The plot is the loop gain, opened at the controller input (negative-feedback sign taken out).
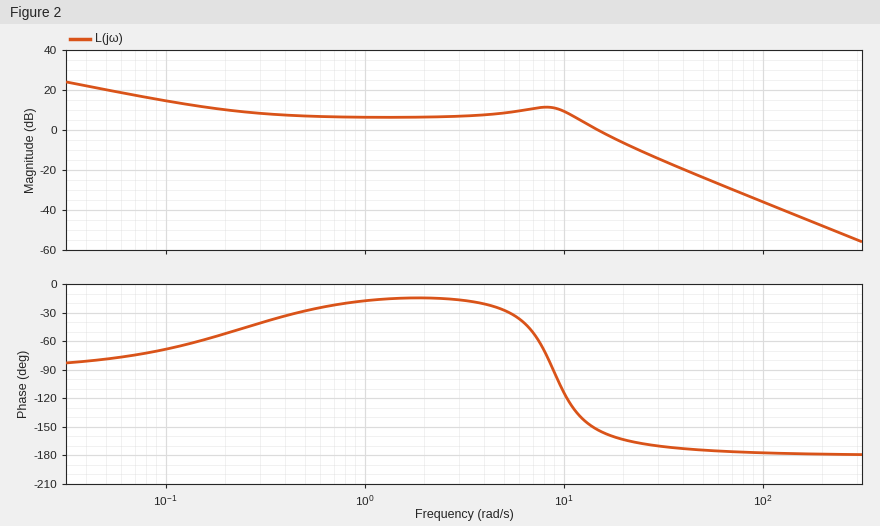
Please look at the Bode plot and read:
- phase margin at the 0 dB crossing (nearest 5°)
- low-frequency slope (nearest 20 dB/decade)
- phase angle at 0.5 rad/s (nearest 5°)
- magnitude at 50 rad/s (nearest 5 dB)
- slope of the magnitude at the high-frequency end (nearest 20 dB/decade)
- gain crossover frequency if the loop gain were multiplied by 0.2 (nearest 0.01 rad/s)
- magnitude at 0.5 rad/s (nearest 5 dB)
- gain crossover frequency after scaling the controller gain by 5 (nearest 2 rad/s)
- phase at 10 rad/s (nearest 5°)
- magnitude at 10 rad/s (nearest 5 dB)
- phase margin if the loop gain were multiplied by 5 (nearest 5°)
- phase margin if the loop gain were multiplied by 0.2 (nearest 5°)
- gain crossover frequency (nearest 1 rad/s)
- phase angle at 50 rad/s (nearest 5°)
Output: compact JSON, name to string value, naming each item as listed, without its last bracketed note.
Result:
{"phase margin at the 0 dB crossing": "25°", "low-frequency slope": "-20 dB/decade", "phase angle at 0.5 rad/s": "-30°", "magnitude at 50 rad/s": "-25 dB", "slope of the magnitude at the high-frequency end": "-40 dB/decade", "gain crossover frequency if the loop gain were multiplied by 0.2": "0.11 rad/s", "magnitude at 0.5 rad/s": "5 dB", "gain crossover frequency after scaling the controller gain by 5": "30 rad/s", "phase at 10 rad/s": "-115°", "magnitude at 10 rad/s": "10 dB", "phase margin if the loop gain were multiplied by 5": "10°", "phase margin if the loop gain were multiplied by 0.2": "115°", "gain crossover frequency": "15 rad/s", "phase angle at 50 rad/s": "-175°"}
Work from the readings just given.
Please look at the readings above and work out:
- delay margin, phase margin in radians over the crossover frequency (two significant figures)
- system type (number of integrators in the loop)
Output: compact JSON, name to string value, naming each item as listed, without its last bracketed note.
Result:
{"delay margin, phase margin in radians over the crossover frequency": "0.029 s", "system type": "1"}
